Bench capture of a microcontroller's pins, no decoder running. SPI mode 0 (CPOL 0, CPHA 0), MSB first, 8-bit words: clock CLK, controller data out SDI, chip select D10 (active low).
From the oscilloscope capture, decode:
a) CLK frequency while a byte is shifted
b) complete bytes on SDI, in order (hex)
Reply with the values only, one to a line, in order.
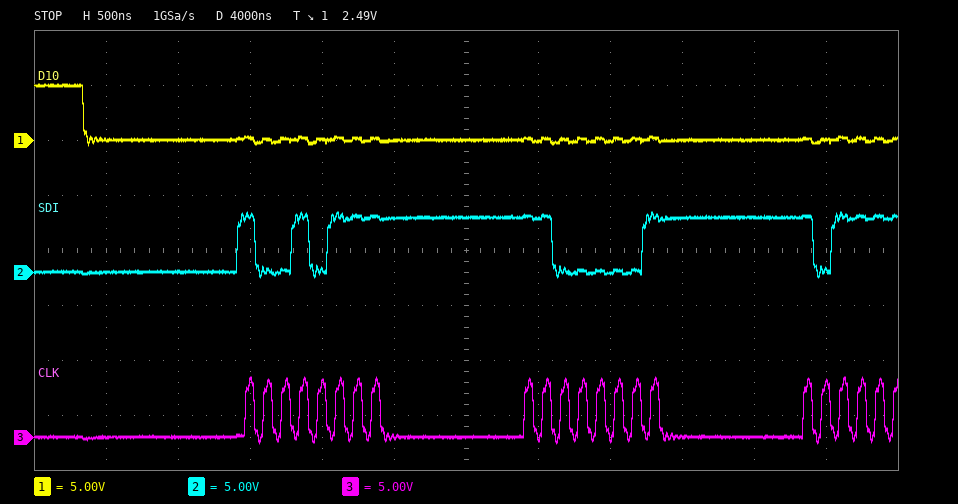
8 MHz
97 C1
